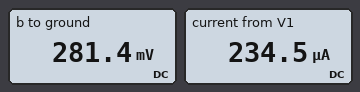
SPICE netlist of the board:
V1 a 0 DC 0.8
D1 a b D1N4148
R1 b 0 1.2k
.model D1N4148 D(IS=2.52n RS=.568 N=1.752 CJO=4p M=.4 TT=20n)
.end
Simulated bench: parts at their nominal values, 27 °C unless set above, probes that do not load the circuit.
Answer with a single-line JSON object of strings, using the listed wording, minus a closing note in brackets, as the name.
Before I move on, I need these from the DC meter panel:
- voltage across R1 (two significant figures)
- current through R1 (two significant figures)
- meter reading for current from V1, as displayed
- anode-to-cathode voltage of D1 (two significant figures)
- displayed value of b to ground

{"voltage across R1": "280 mV", "current through R1": "230 µA", "meter reading for current from V1, as displayed": "234.5 µA", "anode-to-cathode voltage of D1": "520 mV", "displayed value of b to ground": "281.4 mV"}
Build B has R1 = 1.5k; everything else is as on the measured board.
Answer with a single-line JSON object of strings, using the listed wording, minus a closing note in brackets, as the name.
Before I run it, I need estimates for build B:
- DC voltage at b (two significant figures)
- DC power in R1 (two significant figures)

{"DC voltage at b": "290 mV", "DC power in R1": "56 µW"}
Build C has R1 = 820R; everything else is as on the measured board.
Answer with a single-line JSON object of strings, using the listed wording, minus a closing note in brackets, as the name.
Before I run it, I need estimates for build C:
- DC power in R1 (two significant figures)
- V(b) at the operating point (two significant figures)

{"DC power in R1": "87 µW", "V(b) at the operating point": "270 mV"}
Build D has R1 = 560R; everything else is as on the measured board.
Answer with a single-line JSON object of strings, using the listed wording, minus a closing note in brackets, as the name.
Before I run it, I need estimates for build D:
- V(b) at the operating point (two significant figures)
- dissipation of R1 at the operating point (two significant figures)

{"V(b) at the operating point": "250 mV", "dissipation of R1 at the operating point": "110 µW"}
